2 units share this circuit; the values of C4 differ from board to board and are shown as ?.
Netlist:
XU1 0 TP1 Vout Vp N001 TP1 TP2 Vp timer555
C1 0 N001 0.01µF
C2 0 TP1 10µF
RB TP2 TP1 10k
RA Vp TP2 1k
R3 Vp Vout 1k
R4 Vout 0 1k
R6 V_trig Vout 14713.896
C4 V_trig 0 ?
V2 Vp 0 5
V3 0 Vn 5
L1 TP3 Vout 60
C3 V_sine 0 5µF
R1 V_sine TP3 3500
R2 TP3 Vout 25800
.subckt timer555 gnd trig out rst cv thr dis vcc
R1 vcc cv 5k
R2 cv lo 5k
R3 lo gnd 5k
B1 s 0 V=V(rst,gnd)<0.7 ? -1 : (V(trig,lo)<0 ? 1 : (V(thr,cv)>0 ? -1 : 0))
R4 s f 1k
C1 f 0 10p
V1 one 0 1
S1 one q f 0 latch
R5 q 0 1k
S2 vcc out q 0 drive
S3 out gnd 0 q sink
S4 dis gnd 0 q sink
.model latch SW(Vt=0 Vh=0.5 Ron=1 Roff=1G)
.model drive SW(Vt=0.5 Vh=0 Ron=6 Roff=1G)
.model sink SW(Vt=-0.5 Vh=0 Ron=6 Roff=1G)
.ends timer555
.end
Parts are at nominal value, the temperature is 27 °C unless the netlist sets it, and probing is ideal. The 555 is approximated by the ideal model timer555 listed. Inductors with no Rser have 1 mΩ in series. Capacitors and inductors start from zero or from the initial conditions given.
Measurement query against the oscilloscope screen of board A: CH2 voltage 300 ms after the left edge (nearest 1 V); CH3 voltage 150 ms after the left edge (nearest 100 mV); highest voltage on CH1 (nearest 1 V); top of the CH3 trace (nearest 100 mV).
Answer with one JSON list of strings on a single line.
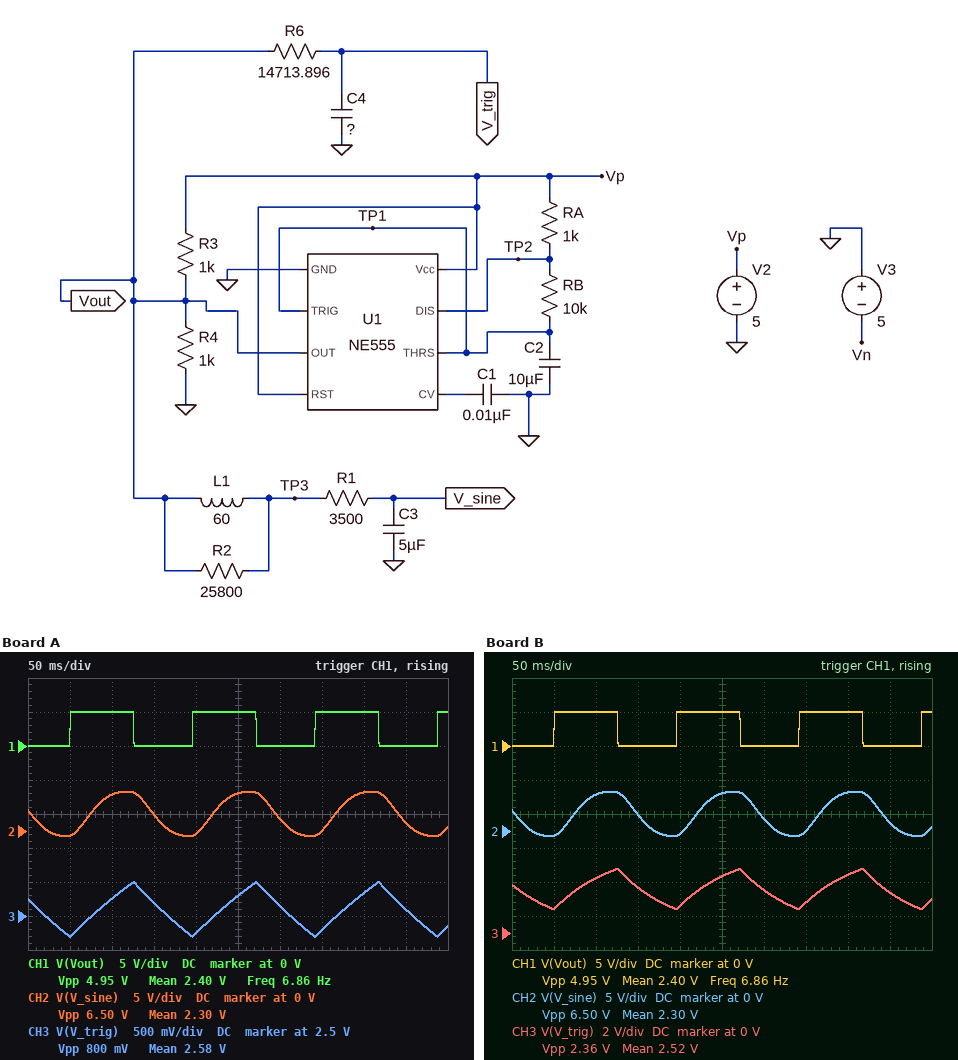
["2 V", "2.7 V", "5 V", "3.0 V"]
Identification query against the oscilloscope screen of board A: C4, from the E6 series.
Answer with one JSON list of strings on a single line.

["15 µF"]
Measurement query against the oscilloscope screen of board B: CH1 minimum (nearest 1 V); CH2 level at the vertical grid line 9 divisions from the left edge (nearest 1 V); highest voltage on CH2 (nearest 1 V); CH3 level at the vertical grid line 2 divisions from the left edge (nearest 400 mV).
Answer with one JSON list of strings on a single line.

["0 V", "1 V", "6 V", "3.2 V"]
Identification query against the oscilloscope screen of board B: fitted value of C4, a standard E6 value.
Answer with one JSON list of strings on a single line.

["4.7 µF"]
